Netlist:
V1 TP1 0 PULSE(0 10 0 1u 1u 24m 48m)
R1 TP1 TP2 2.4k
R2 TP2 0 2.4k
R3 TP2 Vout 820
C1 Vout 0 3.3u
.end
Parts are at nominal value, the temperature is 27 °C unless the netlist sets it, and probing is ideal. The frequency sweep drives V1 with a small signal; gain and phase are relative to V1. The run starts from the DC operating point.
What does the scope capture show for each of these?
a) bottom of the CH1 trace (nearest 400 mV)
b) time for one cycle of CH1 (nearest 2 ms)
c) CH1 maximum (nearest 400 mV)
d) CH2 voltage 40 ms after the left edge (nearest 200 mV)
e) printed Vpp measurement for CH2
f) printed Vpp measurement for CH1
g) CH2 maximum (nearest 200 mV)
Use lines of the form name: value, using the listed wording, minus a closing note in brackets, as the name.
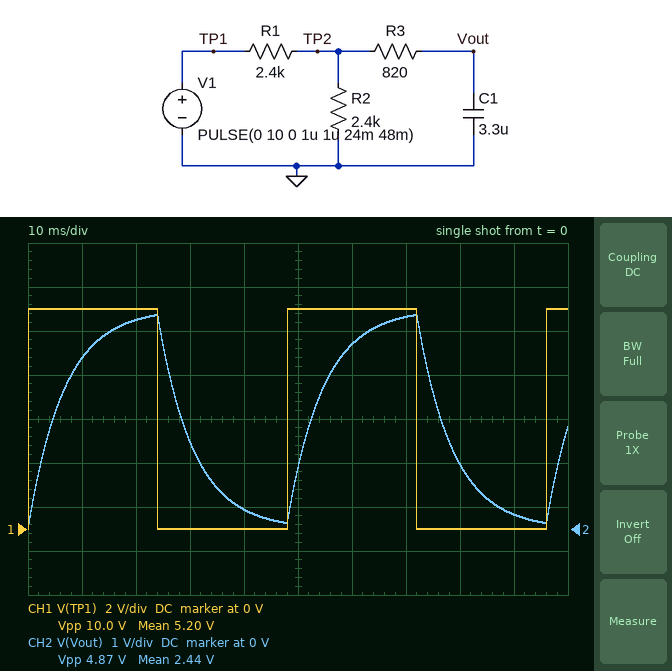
bottom of the CH1 trace: 0 V
time for one cycle of CH1: 48 ms
CH1 maximum: 10.0 V
CH2 voltage 40 ms after the left edge: 400 mV
printed Vpp measurement for CH2: 4.87 V
printed Vpp measurement for CH1: 10.0 V
CH2 maximum: 4.8 V
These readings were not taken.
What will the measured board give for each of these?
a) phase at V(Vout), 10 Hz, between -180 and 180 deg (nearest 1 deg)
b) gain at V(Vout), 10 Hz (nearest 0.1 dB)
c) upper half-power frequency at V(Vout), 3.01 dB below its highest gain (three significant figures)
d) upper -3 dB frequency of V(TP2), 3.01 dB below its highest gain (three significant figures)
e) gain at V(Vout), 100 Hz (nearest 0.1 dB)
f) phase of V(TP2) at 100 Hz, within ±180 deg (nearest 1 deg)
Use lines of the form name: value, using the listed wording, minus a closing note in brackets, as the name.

phase at V(Vout), 10 Hz, between -180 and 180 deg: -23 deg
gain at V(Vout), 10 Hz: -6.7 dB
upper half-power frequency at V(Vout), 3.01 dB below its highest gain: 23.9 Hz
upper -3 dB frequency of V(TP2), 3.01 dB below its highest gain: 29.2 Hz
gain at V(Vout), 100 Hz: -18.7 dB
phase of V(TP2) at 100 Hz, within ±180 deg: -17 deg
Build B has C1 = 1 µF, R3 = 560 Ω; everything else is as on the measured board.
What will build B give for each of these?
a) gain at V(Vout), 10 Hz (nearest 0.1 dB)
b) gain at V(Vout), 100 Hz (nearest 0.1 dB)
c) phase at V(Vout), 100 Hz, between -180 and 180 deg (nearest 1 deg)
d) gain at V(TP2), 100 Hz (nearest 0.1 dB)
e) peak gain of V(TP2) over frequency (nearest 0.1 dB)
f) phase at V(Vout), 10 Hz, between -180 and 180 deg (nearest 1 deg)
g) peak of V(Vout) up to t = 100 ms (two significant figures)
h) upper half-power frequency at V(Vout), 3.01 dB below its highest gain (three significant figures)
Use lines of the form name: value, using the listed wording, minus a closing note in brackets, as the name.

gain at V(Vout), 10 Hz: -6.1 dB
gain at V(Vout), 100 Hz: -9.5 dB
phase at V(Vout), 100 Hz, between -180 and 180 deg: -48 deg
gain at V(TP2), 100 Hz: -9.0 dB
peak gain of V(TP2) over frequency: -6.0 dB
phase at V(Vout), 10 Hz, between -180 and 180 deg: -6 deg
peak of V(Vout) up to t = 100 ms: 5.0 V
upper half-power frequency at V(Vout), 3.01 dB below its highest gain: 90.4 Hz
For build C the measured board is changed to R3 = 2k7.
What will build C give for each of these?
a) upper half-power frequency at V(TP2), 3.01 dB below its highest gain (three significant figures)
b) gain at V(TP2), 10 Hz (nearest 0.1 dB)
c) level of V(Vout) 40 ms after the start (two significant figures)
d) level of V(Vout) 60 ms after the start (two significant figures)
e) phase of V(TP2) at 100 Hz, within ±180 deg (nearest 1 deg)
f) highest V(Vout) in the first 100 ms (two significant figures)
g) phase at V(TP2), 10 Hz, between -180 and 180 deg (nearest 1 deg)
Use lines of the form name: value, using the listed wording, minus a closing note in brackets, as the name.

upper half-power frequency at V(TP2), 3.01 dB below its highest gain: 60.8 Hz
gain at V(TP2), 10 Hz: -7.0 dB
level of V(Vout) 40 ms after the start: 1.2 V
level of V(Vout) 60 ms after the start: 3.3 V
phase of V(TP2) at 100 Hz, within ±180 deg: -3 deg
highest V(Vout) in the first 100 ms: 4.3 V
phase at V(TP2), 10 Hz, between -180 and 180 deg: -10 deg
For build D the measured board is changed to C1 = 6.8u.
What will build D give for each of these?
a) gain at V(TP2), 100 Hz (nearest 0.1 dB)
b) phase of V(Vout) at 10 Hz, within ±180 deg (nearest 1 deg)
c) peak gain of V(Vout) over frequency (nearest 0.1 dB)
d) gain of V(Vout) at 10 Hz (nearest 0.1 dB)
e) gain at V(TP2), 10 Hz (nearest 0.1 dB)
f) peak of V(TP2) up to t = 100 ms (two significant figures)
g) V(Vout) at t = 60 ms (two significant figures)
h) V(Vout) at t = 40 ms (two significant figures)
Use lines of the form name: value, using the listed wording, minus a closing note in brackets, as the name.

gain at V(TP2), 100 Hz: -13.6 dB
phase of V(Vout) at 10 Hz, within ±180 deg: -41 deg
peak gain of V(Vout) over frequency: -6.0 dB
gain of V(Vout) at 10 Hz: -8.4 dB
gain at V(TP2), 10 Hz: -7.9 dB
peak of V(TP2) up to t = 100 ms: 4.6 V
V(Vout) at t = 60 ms: 3.2 V
V(Vout) at t = 40 ms: 1.3 V
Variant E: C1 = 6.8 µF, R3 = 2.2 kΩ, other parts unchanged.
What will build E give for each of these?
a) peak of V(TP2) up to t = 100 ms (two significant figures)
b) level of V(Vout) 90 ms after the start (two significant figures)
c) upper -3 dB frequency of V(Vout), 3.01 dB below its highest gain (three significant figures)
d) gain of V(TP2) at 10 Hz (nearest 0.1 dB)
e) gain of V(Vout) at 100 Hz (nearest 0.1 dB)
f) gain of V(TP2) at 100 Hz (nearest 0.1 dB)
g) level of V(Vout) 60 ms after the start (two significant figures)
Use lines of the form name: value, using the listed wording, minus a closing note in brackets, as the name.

peak of V(TP2) up to t = 100 ms: 4.5 V
level of V(Vout) 90 ms after the start: 1.7 V
upper -3 dB frequency of V(Vout), 3.01 dB below its highest gain: 6.88 Hz
gain of V(TP2) at 10 Hz: -8.2 dB
gain of V(Vout) at 100 Hz: -29.3 dB
gain of V(TP2) at 100 Hz: -9.8 dB
level of V(Vout) 60 ms after the start: 2.7 V
